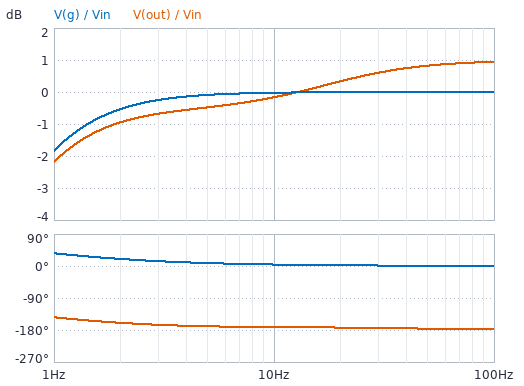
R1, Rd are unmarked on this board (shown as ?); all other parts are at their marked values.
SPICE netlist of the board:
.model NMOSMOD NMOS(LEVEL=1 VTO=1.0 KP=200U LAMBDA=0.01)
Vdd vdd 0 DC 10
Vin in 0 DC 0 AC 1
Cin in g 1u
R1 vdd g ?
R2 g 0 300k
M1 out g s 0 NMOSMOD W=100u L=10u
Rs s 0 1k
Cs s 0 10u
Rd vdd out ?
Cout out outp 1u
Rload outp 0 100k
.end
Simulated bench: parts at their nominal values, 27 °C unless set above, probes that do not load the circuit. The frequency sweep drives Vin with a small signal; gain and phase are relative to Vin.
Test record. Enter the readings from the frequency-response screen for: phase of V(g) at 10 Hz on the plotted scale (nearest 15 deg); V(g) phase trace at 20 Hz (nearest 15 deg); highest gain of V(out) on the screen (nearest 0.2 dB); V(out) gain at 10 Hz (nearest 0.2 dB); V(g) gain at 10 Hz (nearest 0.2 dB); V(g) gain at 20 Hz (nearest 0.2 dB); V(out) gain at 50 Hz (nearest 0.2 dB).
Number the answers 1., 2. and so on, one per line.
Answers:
1. 0 deg
2. 0 deg
3. 1.0 dB
4. -0.2 dB
5. 0 dB
6. 0 dB
7. 0.8 dB
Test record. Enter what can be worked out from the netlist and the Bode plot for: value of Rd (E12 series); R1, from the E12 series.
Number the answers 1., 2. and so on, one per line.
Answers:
1. 12 kΩ
2. 820 kΩ
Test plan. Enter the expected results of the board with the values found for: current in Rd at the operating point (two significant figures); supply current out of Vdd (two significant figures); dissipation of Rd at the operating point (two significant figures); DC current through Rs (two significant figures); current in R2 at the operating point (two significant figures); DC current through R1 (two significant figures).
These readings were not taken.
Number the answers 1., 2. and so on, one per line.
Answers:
1. 730 µA
2. 740 µA
3. 6.4 mW
4. 730 µA
5. 8.9 µA
6. 8.9 µA
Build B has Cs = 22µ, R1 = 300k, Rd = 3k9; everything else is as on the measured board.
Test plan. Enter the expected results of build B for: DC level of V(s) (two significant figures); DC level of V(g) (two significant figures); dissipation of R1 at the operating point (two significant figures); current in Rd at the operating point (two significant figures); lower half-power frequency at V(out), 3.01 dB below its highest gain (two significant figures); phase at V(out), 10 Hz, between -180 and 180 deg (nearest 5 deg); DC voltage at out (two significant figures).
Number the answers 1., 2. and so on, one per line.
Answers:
1. 1.9 V
2. 5.0 V
3. 83 µW
4. 1.9 mA
5. 2.4 Hz
6. -165 deg
7. 2.5 V
